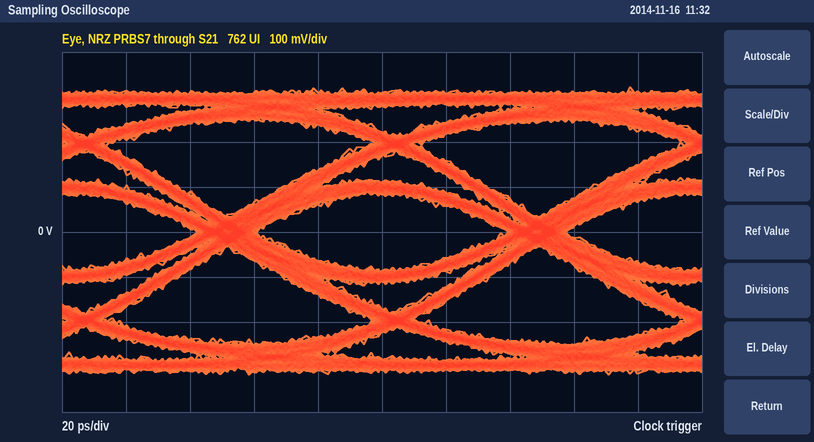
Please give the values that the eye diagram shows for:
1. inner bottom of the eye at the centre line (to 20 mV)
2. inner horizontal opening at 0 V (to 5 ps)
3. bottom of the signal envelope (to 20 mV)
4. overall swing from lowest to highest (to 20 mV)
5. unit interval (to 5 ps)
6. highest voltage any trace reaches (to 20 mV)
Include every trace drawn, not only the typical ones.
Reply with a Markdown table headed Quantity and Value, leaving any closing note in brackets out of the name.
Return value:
| Quantity | Value |
|---|---|
| inner bottom of the eye at the centre line | -80 mV |
| inner horizontal opening at 0 V | 80 ps |
| bottom of the signal envelope | -320 mV |
| overall swing from lowest to highest | 640 mV |
| unit interval | 95 ps |
| highest voltage any trace reaches | 320 mV |
